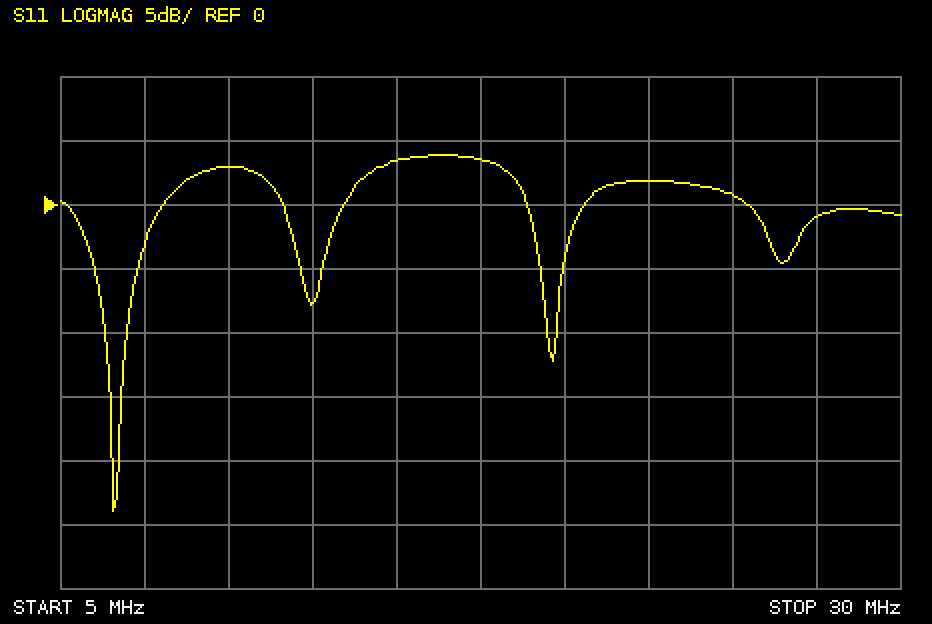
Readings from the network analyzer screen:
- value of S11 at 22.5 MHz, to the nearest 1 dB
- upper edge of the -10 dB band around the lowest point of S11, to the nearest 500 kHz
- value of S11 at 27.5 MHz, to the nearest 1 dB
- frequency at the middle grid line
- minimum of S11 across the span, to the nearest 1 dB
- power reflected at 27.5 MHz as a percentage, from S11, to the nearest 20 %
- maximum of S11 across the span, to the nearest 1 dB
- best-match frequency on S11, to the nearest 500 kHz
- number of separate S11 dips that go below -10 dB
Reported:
2 dB
7.0 MHz
-1 dB
17.5 MHz
-24 dB
80 %
4 dB
6.5 MHz
2
